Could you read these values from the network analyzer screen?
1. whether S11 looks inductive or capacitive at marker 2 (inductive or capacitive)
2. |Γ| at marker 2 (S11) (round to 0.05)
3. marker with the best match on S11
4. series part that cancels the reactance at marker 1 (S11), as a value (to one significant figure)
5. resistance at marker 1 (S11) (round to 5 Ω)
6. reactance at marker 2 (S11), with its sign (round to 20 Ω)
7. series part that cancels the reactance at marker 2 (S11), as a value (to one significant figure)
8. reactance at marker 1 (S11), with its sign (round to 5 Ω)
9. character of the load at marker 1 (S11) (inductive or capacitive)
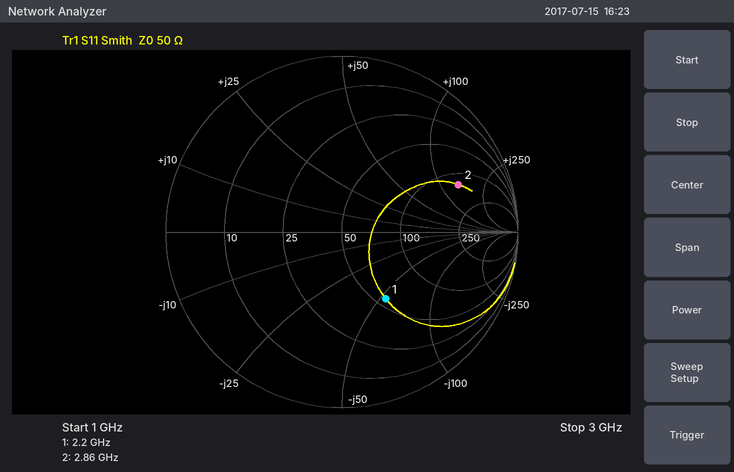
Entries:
inductive
0.70
marker 1
4 nH
55 Ω
+140 Ω
400 fF
-55 Ω
capacitive
